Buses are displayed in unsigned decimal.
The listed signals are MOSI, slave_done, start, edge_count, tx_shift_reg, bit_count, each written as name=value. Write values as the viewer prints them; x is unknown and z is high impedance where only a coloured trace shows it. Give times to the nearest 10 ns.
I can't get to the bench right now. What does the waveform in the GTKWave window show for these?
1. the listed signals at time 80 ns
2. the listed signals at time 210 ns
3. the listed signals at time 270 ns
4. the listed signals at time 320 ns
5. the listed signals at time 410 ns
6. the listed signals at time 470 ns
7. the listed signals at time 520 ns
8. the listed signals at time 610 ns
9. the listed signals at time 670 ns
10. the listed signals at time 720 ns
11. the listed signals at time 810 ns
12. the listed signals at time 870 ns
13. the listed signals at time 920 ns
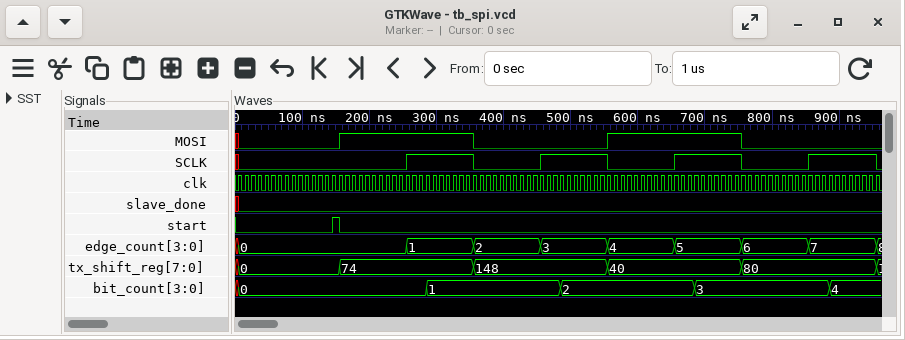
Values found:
MOSI=0, slave_done=0, start=0, edge_count=0, tx_shift_reg=0, bit_count=0
MOSI=1, slave_done=0, start=0, edge_count=0, tx_shift_reg=74, bit_count=0
MOSI=1, slave_done=0, start=0, edge_count=1, tx_shift_reg=74, bit_count=0
MOSI=1, slave_done=0, start=0, edge_count=1, tx_shift_reg=74, bit_count=1
MOSI=0, slave_done=0, start=0, edge_count=2, tx_shift_reg=148, bit_count=1
MOSI=0, slave_done=0, start=0, edge_count=3, tx_shift_reg=148, bit_count=1
MOSI=0, slave_done=0, start=0, edge_count=3, tx_shift_reg=148, bit_count=2
MOSI=1, slave_done=0, start=0, edge_count=4, tx_shift_reg=40, bit_count=2
MOSI=1, slave_done=0, start=0, edge_count=5, tx_shift_reg=40, bit_count=2
MOSI=1, slave_done=0, start=0, edge_count=5, tx_shift_reg=40, bit_count=3
MOSI=0, slave_done=0, start=0, edge_count=6, tx_shift_reg=80, bit_count=3
MOSI=0, slave_done=0, start=0, edge_count=7, tx_shift_reg=80, bit_count=3
MOSI=0, slave_done=0, start=0, edge_count=7, tx_shift_reg=80, bit_count=4
